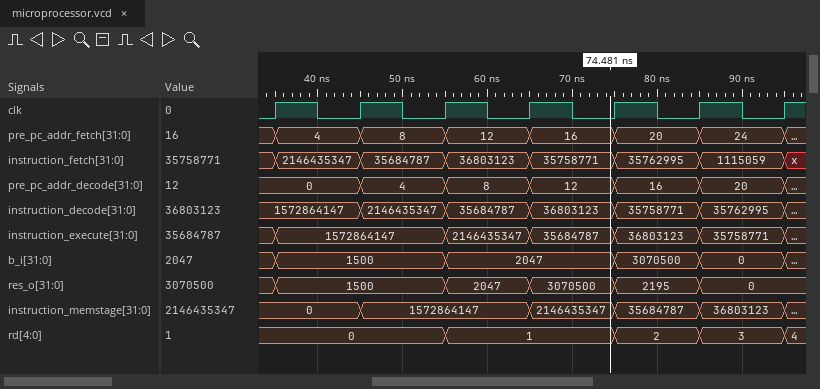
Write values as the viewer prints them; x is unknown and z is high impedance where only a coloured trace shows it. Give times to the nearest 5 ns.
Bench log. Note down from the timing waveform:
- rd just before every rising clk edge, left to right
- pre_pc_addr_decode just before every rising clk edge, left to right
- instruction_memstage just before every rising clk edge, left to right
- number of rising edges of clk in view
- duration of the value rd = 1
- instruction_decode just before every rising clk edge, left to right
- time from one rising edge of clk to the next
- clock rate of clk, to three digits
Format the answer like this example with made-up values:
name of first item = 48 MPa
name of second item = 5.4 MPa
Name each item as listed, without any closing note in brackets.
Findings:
rd just before every rising clk edge, left to right = 0, 0, 0, 1, 1, 2, 3
pre_pc_addr_decode just before every rising clk edge, left to right = 0, 0, 4, 8, 12, 16, 20
instruction_memstage just before every rising clk edge, left to right = 0, 0, 1572864147, 1572864147, 2146435347, 35684787, 36803123
number of rising edges of clk in view = 7
duration of the value rd = 1 = 20 ns
instruction_decode just before every rising clk edge, left to right = 1572864147, 1572864147, 2146435347, 35684787, 36803123, 35758771, 35762995
time from one rising edge of clk to the next = 10 ns
clock rate of clk, to three digits = 100 MHz
